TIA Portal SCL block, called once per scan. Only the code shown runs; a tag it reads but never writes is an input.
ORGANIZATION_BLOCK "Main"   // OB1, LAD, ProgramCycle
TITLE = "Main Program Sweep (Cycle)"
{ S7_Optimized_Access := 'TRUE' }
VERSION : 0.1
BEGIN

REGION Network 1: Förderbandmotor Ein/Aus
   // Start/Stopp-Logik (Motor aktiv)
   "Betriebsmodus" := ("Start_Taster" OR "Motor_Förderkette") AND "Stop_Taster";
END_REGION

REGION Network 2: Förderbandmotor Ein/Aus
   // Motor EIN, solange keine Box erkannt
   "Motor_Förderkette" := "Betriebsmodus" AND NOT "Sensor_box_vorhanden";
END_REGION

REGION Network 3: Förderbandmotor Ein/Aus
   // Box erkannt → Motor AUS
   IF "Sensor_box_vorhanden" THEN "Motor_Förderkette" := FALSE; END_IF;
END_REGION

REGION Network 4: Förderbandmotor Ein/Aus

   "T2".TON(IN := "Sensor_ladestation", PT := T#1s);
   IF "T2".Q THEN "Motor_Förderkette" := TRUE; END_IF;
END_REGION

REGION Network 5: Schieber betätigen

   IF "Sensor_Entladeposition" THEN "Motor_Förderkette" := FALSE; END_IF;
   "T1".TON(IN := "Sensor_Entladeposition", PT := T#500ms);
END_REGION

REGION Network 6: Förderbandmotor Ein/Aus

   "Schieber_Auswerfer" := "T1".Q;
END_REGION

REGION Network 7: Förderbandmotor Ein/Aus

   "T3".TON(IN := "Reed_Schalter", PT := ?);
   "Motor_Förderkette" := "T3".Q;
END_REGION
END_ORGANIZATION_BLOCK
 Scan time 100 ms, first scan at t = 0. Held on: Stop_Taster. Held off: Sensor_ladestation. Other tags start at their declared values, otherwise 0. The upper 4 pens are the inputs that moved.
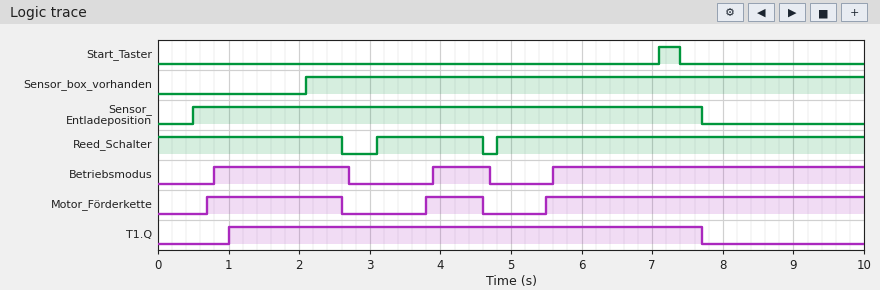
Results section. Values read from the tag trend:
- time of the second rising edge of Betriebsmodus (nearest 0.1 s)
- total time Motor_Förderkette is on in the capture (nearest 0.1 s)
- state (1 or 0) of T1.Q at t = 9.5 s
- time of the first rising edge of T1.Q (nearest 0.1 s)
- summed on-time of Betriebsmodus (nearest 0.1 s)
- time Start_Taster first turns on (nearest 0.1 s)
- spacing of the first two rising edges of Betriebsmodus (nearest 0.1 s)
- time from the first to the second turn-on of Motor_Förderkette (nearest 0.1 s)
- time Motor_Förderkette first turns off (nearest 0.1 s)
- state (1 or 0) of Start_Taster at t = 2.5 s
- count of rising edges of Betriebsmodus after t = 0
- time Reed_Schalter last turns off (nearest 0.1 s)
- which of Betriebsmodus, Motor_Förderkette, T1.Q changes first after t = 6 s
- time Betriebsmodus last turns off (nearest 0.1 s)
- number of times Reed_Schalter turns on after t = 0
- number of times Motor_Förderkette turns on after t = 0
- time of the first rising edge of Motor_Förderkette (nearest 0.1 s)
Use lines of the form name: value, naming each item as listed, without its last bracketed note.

time of the second rising edge of Betriebsmodus: 3.9 s
total time Motor_Förderkette is on in the capture: 7.2 s
state (1 or 0) of T1.Q at t = 9.5 s: 0
time of the first rising edge of T1.Q: 1.0 s
summed on-time of Betriebsmodus: 7.1 s
time Start_Taster first turns on: 7.1 s
spacing of the first two rising edges of Betriebsmodus: 3.1 s
time from the first to the second turn-on of Motor_Förderkette: 3.1 s
time Motor_Förderkette first turns off: 2.6 s
state (1 or 0) of Start_Taster at t = 2.5 s: 0
count of rising edges of Betriebsmodus after t = 0: 3
time Reed_Schalter last turns off: 4.6 s
which of Betriebsmodus, Motor_Förderkette, T1.Q changes first after t = 6 s: T1.Q
time Betriebsmodus last turns off: 4.7 s
number of times Reed_Schalter turns on after t = 0: 2
number of times Motor_Förderkette turns on after t = 0: 3
time of the first rising edge of Motor_Förderkette: 0.7 s
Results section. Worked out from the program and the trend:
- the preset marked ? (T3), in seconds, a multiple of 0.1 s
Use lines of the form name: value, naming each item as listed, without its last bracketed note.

the preset marked ? (T3), in seconds, a multiple of 0.1 s: 0.7 s
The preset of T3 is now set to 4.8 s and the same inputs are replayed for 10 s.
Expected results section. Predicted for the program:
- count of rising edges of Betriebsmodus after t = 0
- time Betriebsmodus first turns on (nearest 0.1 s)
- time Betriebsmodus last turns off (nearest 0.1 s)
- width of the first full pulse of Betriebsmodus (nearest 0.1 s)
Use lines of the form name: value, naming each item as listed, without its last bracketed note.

count of rising edges of Betriebsmodus after t = 0: 2
time Betriebsmodus first turns on: 7.1 s
time Betriebsmodus last turns off: 7.4 s
width of the first full pulse of Betriebsmodus: 0.3 s
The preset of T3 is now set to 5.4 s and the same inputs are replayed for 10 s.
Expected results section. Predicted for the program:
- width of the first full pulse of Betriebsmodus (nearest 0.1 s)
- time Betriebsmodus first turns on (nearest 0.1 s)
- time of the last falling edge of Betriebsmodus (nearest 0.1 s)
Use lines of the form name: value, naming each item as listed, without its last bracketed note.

width of the first full pulse of Betriebsmodus: 0.3 s
time Betriebsmodus first turns on: 7.1 s
time of the last falling edge of Betriebsmodus: 7.4 s
